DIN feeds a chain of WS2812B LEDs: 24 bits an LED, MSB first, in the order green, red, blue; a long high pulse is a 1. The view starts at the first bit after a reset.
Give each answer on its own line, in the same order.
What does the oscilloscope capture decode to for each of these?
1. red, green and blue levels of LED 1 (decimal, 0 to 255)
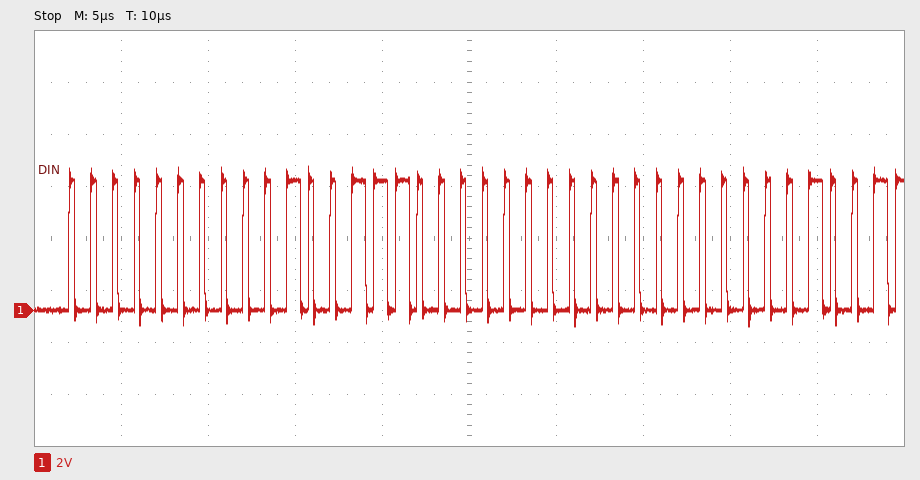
39, 0, 0
